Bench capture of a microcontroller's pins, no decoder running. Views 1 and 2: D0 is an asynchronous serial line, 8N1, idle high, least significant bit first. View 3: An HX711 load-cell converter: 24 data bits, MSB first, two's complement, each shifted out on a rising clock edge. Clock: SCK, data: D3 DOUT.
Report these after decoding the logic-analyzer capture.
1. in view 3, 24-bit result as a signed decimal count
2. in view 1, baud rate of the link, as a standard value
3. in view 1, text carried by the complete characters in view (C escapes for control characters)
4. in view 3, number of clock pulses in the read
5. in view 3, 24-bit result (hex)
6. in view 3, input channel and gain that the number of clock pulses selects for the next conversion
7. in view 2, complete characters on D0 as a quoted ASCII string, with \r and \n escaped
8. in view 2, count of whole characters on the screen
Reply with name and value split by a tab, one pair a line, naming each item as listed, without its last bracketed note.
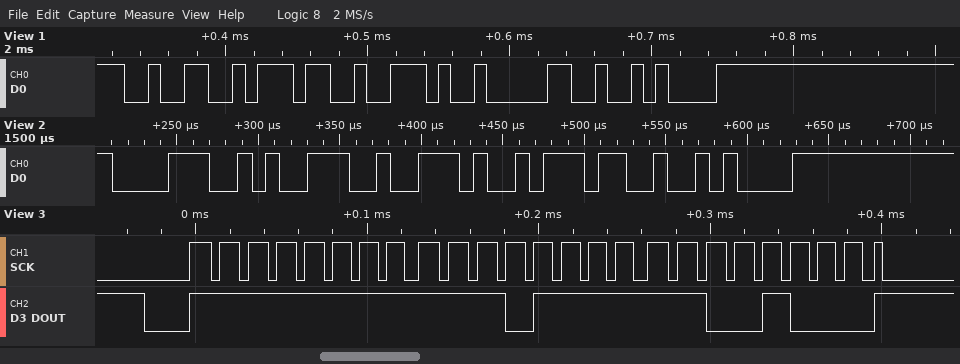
in view 3, 24-bit result as a signed decimal count	-4152
in view 1, baud rate of the link, as a standard value	115200 baud
in view 1, text carried by the complete characters in view	"27.0\n"
in view 3, number of clock pulses in the read	25
in view 3, 24-bit result	0xFFEFC8
in view 3, input channel and gain that the number of clock pulses selects for the next conversion	channel A, gain 128
in view 2, complete characters on D0 as a quoted ASCII string, with \r and \n escaped	"89.7\n"
in view 2, count of whole characters on the screen	5
